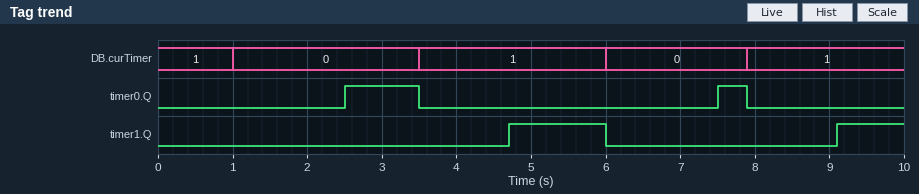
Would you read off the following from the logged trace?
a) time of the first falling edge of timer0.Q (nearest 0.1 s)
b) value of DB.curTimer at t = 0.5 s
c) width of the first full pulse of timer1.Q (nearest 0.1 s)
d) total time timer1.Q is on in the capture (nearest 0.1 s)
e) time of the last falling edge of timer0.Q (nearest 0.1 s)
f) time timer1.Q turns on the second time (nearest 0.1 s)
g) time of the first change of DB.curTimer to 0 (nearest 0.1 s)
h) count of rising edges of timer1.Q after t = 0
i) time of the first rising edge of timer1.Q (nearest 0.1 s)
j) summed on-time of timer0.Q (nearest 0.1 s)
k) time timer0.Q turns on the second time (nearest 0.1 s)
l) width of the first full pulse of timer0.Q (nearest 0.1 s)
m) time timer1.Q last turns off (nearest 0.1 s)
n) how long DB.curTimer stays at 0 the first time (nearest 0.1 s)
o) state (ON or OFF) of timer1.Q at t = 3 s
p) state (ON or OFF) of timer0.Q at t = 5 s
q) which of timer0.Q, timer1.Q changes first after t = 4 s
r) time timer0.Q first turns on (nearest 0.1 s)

3.5 s
1
1.3 s
2.2 s
7.9 s
9.1 s
1.0 s
2
4.7 s
1.4 s
7.5 s
1.0 s
6.0 s
2.5 s
OFF
OFF
timer1.Q
2.5 s
